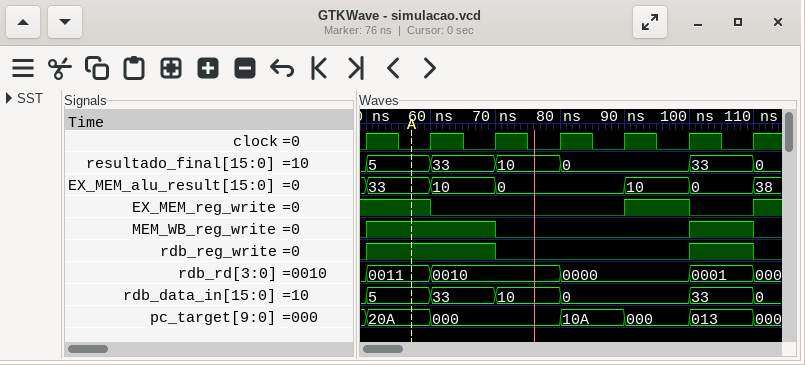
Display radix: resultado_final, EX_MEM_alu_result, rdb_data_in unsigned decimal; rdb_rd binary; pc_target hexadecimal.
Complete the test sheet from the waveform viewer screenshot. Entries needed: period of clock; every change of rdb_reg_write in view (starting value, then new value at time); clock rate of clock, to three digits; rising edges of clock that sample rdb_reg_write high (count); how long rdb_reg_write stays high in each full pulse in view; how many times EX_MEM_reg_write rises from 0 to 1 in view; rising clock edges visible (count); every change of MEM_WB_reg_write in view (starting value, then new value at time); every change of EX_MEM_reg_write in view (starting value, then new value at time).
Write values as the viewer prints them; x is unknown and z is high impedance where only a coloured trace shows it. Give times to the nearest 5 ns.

10 ns
0, 1 at 50 ns, 0 at 70 ns, 1 at 100 ns, 0 at 110 ns
100 MHz
3
20 ns, 10 ns
2
7
0, 1 at 50 ns, 0 at 70 ns, 1 at 100 ns, 0 at 110 ns
1, 0 at 60 ns, 1 at 90 ns, 0 at 100 ns, 1 at 110 ns
